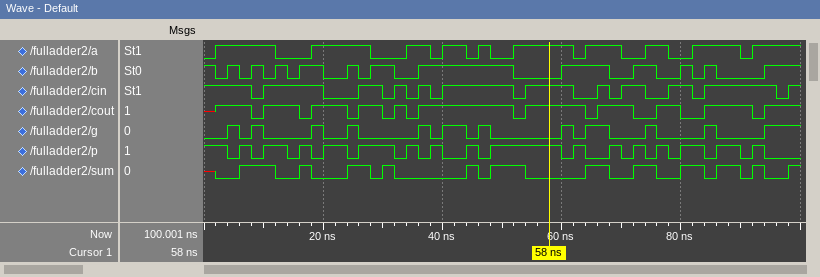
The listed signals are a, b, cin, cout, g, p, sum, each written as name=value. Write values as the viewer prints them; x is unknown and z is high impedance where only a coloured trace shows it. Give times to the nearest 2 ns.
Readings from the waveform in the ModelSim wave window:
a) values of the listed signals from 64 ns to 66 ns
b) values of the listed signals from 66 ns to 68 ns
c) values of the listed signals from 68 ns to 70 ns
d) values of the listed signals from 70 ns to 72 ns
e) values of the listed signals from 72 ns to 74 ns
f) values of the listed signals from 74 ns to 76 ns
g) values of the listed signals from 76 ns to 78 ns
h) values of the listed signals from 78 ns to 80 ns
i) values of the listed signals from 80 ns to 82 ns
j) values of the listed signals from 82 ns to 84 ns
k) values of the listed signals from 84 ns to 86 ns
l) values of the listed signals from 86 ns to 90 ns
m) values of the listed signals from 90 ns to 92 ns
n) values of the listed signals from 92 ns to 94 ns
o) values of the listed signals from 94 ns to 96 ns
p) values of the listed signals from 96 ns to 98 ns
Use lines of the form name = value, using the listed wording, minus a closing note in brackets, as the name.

values of the listed signals from 64 ns to 66 ns = a=1, b=1, cin=0, cout=0, g=1, p=0, sum=1
values of the listed signals from 66 ns to 68 ns = a=1, b=1, cin=1, cout=1, g=1, p=0, sum=1
values of the listed signals from 68 ns to 70 ns = a=1, b=0, cin=0, cout=1, g=0, p=1, sum=0
values of the listed signals from 70 ns to 72 ns = a=0, b=0, cin=1, cout=1, g=0, p=0, sum=0
values of the listed signals from 72 ns to 74 ns = a=0, b=1, cin=1, cout=0, g=0, p=1, sum=1
values of the listed signals from 74 ns to 76 ns = a=1, b=1, cin=0, cout=0, g=1, p=0, sum=1
values of the listed signals from 76 ns to 78 ns = a=1, b=0, cin=0, cout=1, g=0, p=1, sum=0
values of the listed signals from 78 ns to 80 ns = a=0, b=0, cin=1, cout=1, g=0, p=0, sum=0
values of the listed signals from 80 ns to 82 ns = a=0, b=1, cin=1, cout=0, g=0, p=1, sum=1
values of the listed signals from 82 ns to 84 ns = a=1, b=0, cin=0, cout=0, g=0, p=1, sum=1
values of the listed signals from 84 ns to 86 ns = a=1, b=1, cin=1, cout=1, g=1, p=0, sum=0
values of the listed signals from 86 ns to 90 ns = a=1, b=0, cin=1, cout=1, g=0, p=1, sum=1
values of the listed signals from 90 ns to 92 ns = a=0, b=0, cin=1, cout=1, g=0, p=0, sum=0
values of the listed signals from 92 ns to 94 ns = a=1, b=0, cin=1, cout=0, g=0, p=1, sum=1
values of the listed signals from 94 ns to 96 ns = a=1, b=1, cin=1, cout=1, g=1, p=0, sum=0
values of the listed signals from 96 ns to 98 ns = a=1, b=1, cin=0, cout=1, g=1, p=0, sum=0
